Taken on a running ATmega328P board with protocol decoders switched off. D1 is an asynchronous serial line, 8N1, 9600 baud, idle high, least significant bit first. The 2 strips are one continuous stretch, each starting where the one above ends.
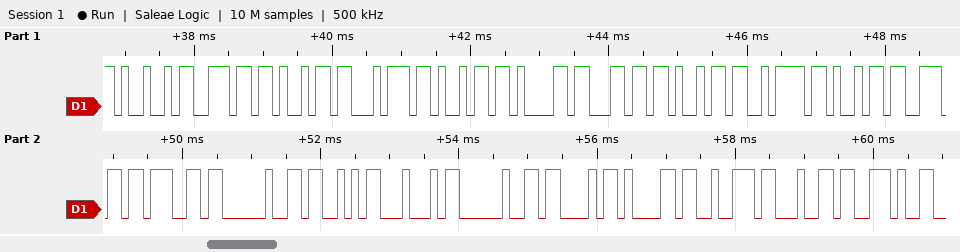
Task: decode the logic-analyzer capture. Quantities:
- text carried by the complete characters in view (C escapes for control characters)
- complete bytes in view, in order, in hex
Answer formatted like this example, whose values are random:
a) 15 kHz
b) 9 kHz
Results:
a) "Initializing SD Card."
b) 0x49 0x6E 0x69 0x74 0x69 0x61 0x6C 0x69 0x7A 0x69 0x6E 0x67 0x20 0x53 0x44 0x20 0x43 0x61 0x72 0x64 0x2E
